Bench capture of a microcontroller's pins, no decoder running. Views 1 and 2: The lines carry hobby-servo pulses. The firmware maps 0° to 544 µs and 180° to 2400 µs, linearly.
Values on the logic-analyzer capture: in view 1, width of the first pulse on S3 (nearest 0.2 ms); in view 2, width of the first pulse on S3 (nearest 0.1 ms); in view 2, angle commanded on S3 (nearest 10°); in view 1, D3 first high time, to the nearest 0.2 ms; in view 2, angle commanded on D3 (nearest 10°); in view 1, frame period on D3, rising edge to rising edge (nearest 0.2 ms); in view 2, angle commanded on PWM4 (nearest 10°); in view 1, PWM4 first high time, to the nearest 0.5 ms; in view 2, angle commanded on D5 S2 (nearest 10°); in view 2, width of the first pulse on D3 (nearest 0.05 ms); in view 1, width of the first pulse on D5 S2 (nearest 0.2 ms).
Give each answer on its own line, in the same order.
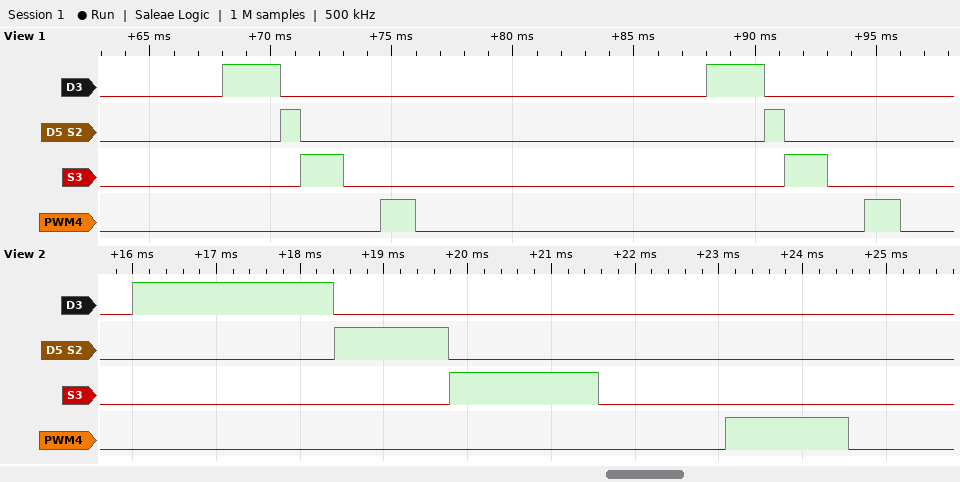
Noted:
1.8 ms
1.8 ms
120°
2.4 ms
180°
20.0 ms
90°
1.5 ms
80°
2.40 ms
0.8 ms
